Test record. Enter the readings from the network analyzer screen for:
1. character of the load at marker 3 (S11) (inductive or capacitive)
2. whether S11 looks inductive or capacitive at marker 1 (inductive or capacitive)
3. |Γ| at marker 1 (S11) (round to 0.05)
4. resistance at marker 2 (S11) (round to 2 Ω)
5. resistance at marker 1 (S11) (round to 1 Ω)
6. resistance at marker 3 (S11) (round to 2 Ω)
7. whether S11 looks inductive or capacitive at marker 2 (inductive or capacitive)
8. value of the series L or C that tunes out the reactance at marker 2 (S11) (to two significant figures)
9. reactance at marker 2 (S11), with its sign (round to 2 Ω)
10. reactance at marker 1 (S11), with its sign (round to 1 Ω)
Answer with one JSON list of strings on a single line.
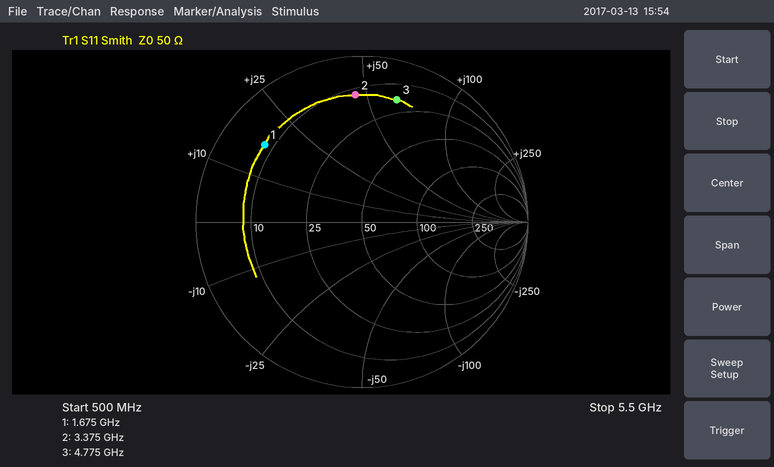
["inductive", "inductive", "0.75", "12 Ω", "8 Ω", "18 Ω", "inductive", "1.0 pF", "+46 Ω", "+17 Ω"]
